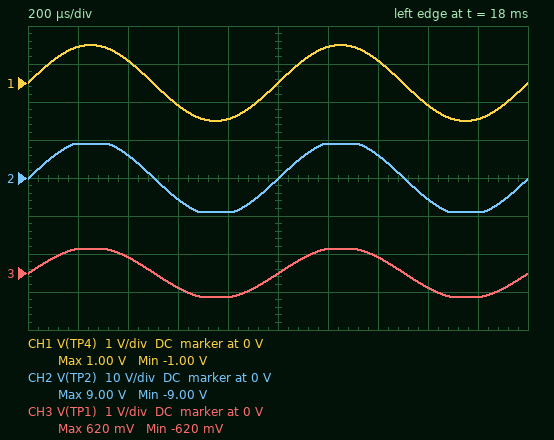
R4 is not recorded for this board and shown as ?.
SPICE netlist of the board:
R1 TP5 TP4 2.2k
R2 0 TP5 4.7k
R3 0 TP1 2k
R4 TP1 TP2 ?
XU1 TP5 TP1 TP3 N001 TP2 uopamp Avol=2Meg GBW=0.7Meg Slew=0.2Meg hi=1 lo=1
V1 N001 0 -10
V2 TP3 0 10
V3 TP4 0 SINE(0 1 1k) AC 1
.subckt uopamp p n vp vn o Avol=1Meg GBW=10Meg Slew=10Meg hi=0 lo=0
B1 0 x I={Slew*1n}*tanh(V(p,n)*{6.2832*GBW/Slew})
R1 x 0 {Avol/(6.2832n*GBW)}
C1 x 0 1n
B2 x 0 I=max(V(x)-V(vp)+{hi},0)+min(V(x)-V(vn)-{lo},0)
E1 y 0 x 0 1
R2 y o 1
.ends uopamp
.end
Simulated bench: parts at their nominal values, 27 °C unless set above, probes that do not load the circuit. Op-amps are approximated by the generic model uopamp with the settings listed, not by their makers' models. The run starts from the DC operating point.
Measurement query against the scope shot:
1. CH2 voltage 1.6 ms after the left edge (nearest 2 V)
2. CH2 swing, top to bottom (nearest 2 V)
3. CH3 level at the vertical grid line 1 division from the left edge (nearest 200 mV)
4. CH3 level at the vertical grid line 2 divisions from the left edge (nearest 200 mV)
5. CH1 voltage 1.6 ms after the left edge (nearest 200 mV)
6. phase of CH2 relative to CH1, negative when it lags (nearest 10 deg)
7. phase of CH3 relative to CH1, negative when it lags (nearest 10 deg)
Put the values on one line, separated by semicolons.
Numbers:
-6 V; 18 V; 600 mV; 400 mV; -600 mV; 0 deg; 0 deg
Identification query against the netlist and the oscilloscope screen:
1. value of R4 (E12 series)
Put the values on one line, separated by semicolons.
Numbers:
27 kΩ
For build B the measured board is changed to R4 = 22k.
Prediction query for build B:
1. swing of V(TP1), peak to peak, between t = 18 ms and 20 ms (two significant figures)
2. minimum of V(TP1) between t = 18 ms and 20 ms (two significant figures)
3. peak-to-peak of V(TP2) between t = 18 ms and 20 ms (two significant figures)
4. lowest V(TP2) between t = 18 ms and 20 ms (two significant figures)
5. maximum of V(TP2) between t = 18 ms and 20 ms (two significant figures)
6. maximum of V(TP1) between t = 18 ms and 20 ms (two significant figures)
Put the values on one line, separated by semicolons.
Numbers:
1.4 V; -680 mV; 16 V; -8.2 V; 8.2 V; 680 mV
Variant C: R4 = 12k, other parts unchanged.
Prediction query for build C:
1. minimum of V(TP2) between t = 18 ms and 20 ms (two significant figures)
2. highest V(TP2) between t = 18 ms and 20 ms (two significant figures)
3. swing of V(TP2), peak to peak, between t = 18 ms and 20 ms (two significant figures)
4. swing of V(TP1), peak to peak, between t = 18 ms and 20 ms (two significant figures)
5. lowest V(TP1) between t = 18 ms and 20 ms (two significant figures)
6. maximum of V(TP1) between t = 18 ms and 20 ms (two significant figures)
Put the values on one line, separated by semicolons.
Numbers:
-4.8 V; 4.8 V; 9.5 V; 1.4 V; -680 mV; 680 mV
